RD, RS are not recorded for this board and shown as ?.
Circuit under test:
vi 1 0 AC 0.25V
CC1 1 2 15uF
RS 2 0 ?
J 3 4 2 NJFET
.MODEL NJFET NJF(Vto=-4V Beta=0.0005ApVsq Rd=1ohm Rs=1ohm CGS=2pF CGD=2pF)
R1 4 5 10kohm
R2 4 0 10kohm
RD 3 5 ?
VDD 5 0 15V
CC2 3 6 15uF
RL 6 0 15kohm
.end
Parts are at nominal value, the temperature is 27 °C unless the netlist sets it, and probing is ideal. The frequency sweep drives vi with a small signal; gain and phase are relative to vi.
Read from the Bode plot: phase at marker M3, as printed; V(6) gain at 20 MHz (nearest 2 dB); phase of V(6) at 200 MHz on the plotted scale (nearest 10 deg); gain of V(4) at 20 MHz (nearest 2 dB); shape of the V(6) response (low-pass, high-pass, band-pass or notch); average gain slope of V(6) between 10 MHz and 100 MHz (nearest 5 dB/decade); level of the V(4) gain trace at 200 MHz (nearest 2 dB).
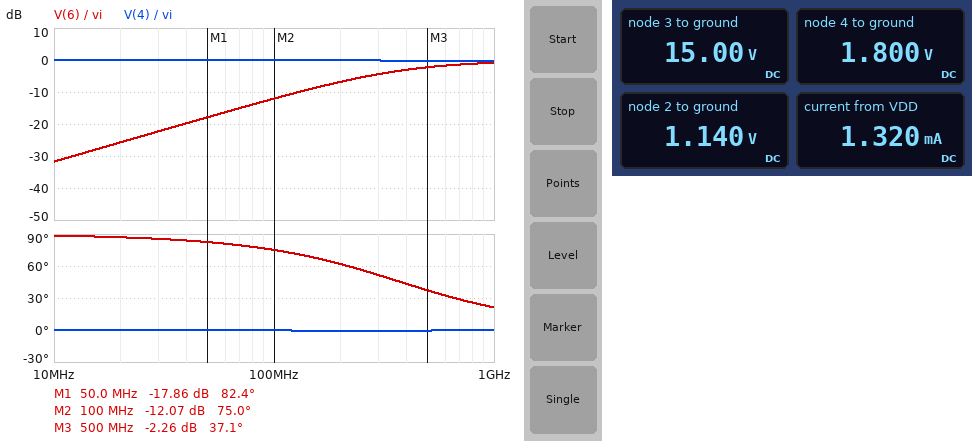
37.1 deg
-26 dB
60 deg
0 dB
high-pass
20 dB/decade
0 dB
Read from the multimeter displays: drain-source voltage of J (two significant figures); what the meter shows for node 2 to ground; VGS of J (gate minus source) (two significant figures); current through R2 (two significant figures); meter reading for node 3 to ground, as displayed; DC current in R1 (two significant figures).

14 V
1.140 V
660 mV
180 µA
15.00 V
1.3 mA
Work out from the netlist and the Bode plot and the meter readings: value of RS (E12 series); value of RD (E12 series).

1 kΩ
820 Ω
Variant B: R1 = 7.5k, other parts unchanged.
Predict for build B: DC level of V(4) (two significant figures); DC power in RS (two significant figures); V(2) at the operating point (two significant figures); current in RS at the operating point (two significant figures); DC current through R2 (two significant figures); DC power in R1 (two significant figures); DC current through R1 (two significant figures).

2.2 V
2.2 mW
1.5 V
1.5 mA
220 µA
22 mW
1.7 mA
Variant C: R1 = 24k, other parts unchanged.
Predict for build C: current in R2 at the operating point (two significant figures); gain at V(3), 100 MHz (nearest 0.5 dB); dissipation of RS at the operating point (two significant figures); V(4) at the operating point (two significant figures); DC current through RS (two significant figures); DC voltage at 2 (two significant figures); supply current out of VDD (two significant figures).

110 µA
-12.5 dB
220 µW
1.1 V
470 µA
470 mV
580 µA
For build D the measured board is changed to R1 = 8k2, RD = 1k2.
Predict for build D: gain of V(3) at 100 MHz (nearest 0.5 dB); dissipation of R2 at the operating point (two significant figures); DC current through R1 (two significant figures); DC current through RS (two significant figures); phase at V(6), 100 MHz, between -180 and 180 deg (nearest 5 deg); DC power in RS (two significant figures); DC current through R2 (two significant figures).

-9.0 dB
420 µW
1.6 mA
1.4 mA
70 deg
1.9 mW
200 µA
